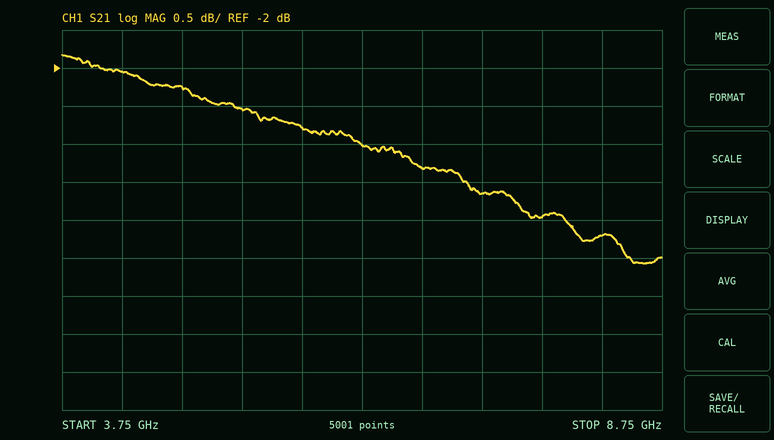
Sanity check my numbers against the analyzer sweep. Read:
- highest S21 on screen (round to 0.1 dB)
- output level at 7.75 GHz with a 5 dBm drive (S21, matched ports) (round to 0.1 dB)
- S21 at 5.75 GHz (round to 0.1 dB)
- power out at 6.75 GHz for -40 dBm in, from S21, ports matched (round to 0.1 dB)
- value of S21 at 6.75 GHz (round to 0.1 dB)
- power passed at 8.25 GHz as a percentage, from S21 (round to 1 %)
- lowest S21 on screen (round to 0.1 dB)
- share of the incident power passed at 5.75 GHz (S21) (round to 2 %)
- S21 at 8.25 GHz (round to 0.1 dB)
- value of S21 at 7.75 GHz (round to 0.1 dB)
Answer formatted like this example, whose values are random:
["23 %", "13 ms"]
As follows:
["-1.8 dB", "1.0 dBm", "-2.8 dB", "-43.3 dBm", "-3.3 dB", "38 %", "-4.6 dB", "52 %", "-4.2 dB", "-4.0 dB"]
